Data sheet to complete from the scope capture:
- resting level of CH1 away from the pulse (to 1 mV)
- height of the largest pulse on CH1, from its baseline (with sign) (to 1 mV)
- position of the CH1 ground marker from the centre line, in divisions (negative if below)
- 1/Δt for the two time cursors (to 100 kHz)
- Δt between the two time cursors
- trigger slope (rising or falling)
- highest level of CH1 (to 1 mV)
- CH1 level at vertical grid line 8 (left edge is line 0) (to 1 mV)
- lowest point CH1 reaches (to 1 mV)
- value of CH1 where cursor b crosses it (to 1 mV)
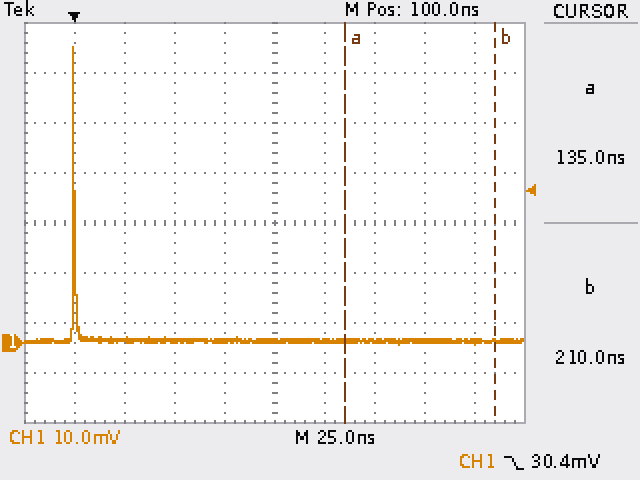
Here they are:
0 mV
+59 mV
-2.4 div
13.3 MHz
75.0 ns
falling
59 mV
0 mV
0 mV
0 mV
